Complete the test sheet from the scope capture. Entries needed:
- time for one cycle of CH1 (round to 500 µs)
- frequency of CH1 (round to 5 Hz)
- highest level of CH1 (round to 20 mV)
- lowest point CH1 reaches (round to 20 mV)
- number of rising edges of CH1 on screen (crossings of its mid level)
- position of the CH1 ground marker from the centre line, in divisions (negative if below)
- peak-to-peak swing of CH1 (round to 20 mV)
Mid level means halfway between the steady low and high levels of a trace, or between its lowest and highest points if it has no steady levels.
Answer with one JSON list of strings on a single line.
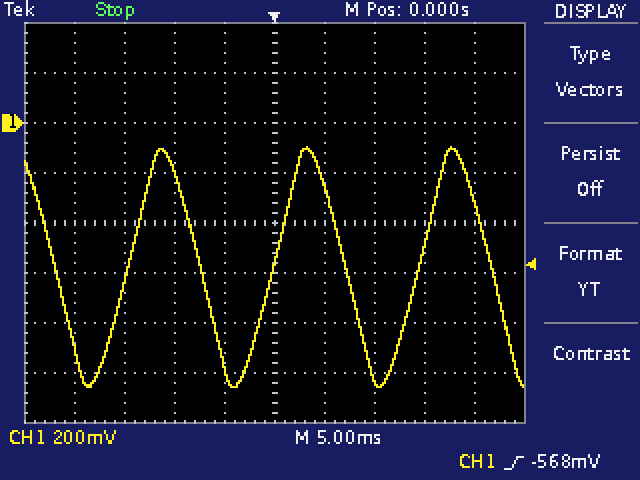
["14.5 ms", "70 Hz", "-100 mV", "-1.06 V", "3", "+2.0 div", "960 mV"]
